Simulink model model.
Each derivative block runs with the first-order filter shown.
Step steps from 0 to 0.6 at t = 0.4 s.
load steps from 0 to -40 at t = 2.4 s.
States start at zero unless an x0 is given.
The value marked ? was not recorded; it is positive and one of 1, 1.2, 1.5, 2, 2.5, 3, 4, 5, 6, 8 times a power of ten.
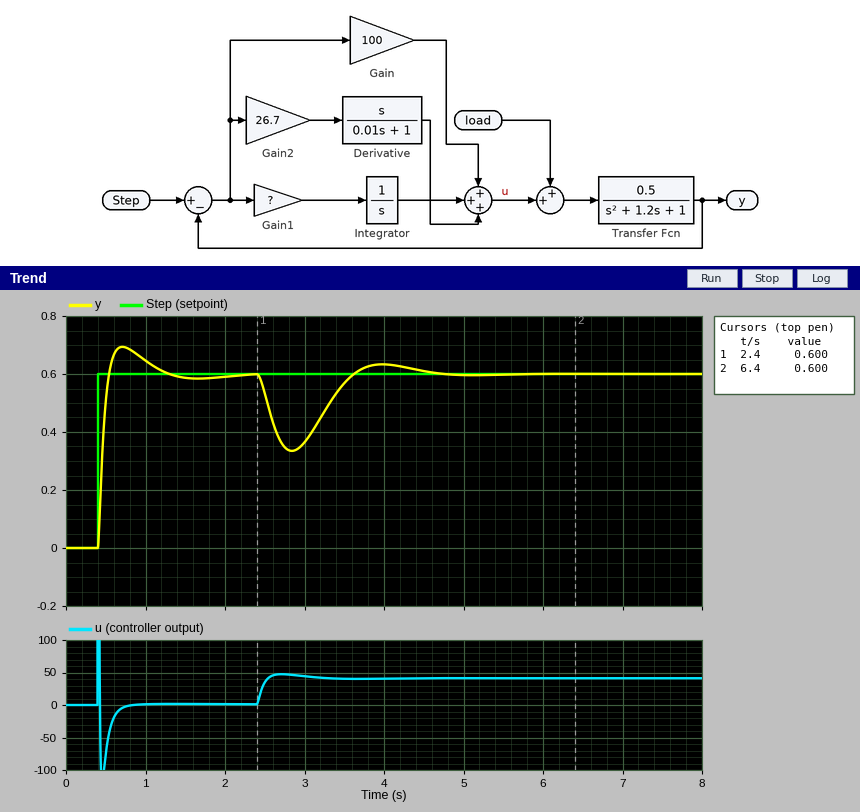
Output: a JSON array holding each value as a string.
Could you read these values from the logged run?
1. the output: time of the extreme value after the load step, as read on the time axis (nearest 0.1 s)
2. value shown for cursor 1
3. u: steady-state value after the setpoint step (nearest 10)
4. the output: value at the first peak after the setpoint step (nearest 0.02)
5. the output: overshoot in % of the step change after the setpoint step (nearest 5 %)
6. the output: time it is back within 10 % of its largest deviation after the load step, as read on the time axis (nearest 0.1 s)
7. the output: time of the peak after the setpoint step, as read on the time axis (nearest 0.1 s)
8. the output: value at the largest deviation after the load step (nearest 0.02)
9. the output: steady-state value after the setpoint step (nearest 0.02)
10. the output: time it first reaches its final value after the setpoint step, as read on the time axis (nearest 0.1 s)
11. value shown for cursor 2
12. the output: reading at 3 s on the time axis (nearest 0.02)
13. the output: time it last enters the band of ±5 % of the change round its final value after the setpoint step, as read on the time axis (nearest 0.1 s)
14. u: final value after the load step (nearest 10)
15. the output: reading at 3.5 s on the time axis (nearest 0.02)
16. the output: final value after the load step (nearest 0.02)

["2.8 s", "0.600", "0", "0.70", "15 %", "4.2 s", "0.7 s", "0.34", "0.60", "0.5 s", "0.600", "0.36", "1.1 s", "40", "0.56", "0.60"]
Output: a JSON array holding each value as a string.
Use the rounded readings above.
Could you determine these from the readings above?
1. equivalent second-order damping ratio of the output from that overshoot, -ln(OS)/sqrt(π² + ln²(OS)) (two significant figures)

["0.52"]
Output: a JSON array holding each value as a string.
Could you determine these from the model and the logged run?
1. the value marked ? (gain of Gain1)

["250"]
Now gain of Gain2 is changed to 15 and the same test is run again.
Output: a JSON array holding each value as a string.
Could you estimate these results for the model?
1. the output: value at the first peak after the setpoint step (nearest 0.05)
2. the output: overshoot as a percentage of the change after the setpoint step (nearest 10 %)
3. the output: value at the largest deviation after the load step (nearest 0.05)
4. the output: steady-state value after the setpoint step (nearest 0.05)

["0.80", "30 %", "0.25", "0.60"]
